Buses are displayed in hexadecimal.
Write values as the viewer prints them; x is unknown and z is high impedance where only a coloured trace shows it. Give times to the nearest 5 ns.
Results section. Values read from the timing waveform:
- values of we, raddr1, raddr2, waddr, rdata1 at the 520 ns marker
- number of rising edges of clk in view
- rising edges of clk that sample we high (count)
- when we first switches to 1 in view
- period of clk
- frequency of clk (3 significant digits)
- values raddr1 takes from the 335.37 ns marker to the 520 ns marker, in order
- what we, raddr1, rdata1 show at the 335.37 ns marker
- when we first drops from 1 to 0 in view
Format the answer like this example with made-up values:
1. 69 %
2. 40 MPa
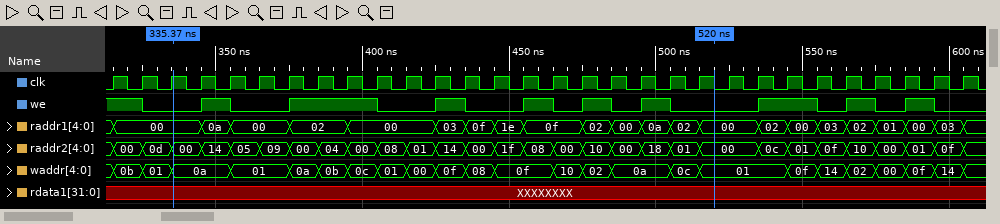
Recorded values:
1. we=0, raddr1=00, raddr2=00, waddr=01, rdata1=XXXXXXXX
2. 30
3. 14
4. 345 ns
5. 10 ns
6. 100 MHz
7. 00, 0a, 00, 02, 00, 03, 0f, 1e, 0f, 02, 00, 0a, 02, 00
8. we=0, raddr1=00, rdata1=XXXXXXXX
9. 325 ns
